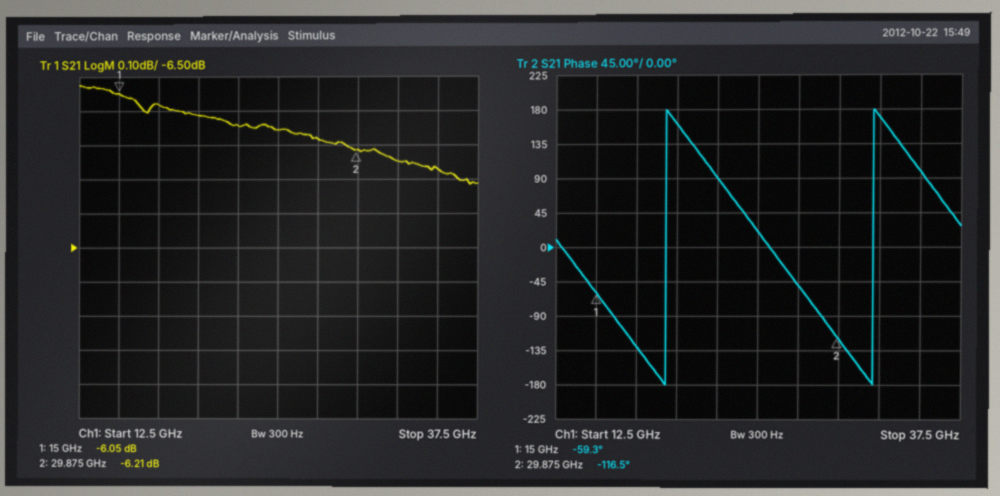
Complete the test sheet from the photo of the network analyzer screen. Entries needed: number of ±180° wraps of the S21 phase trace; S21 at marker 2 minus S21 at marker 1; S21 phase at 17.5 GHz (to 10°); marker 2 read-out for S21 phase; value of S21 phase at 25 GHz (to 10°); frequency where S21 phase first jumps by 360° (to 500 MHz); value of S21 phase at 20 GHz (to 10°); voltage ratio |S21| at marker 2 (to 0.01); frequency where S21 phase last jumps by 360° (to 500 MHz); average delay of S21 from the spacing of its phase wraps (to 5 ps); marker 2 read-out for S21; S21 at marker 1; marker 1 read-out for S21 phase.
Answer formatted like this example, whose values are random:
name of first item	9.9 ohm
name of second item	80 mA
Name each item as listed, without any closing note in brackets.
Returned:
number of ±180° wraps of the S21 phase trace	2
S21 at marker 2 minus S21 at marker 1	-0.16 dB
S21 phase at 17.5 GHz	-130°
marker 2 read-out for S21 phase	-116.5°
value of S21 phase at 25 GHz	20°
frequency where S21 phase first jumps by 360°	19.5 GHz
value of S21 phase at 20 GHz	160°
voltage ratio |S21| at marker 2	0.49
frequency where S21 phase last jumps by 360°	32.0 GHz
average delay of S21 from the spacing of its phase wraps	80 ps
marker 2 read-out for S21	-6.21 dB
S21 at marker 1	-6.05 dB
marker 1 read-out for S21 phase	-59.3°
